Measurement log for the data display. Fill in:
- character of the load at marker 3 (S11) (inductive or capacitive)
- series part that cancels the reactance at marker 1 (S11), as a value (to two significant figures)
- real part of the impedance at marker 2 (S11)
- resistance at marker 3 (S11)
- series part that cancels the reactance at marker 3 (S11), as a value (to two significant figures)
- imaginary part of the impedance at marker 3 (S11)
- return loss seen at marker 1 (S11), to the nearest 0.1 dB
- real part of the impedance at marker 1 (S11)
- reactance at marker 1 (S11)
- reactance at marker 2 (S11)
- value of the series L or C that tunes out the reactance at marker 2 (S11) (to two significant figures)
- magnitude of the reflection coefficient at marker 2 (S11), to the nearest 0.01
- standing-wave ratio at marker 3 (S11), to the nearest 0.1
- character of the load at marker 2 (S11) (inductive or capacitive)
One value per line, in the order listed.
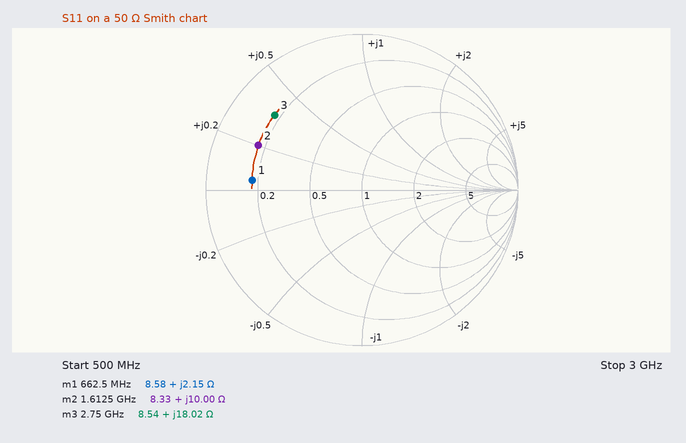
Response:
inductive
110 pF
8.33 Ω
8.54 Ω
3.2 pF
+18.02 Ω
3.0 dB
8.58 Ω
+2.15 Ω
+10.00 Ω
9.9 pF
0.72
6.6
inductive
